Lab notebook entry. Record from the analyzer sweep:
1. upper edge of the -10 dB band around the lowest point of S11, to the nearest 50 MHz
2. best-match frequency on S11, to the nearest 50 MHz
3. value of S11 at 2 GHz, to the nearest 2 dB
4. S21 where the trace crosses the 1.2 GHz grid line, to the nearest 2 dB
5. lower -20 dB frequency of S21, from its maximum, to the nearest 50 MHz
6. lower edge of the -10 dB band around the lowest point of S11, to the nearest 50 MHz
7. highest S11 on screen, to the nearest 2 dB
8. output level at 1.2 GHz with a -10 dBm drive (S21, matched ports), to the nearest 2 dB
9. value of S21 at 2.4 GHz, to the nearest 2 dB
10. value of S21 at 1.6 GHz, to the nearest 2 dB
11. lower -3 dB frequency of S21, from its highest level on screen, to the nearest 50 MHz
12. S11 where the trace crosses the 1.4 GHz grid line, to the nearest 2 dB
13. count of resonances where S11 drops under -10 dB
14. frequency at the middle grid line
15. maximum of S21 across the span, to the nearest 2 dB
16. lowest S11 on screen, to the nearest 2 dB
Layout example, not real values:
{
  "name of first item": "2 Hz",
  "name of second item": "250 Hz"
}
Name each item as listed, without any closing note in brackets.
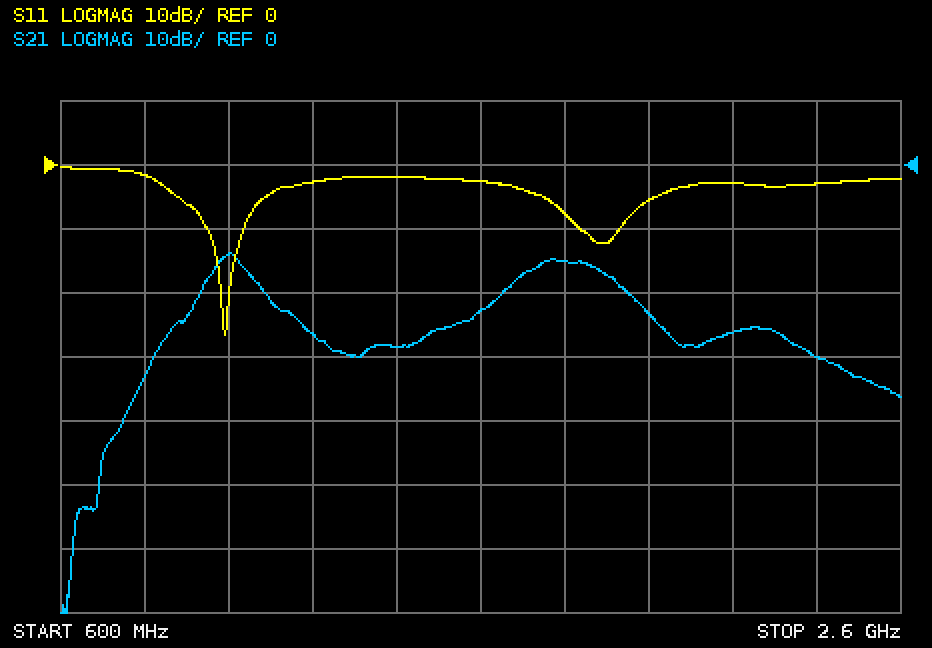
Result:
{
  "upper edge of the -10 dB band around the lowest point of S11, to the nearest 50 MHz": "1.05 GHz",
  "best-match frequency on S11, to the nearest 50 MHz": "1.00 GHz",
  "value of S11 at 2 GHz, to the nearest 2 dB": "-6 dB",
  "S21 where the trace crosses the 1.2 GHz grid line, to the nearest 2 dB": "-26 dB",
  "lower -20 dB frequency of S21, from its maximum, to the nearest 50 MHz": "800 MHz",
  "lower edge of the -10 dB band around the lowest point of S11, to the nearest 50 MHz": "950 MHz",
  "highest S11 on screen, to the nearest 2 dB": "0 dB",
  "output level at 1.2 GHz with a -10 dBm drive (S21, matched ports), to the nearest 2 dB": "-36 dBm",
  "value of S21 at 2.4 GHz, to the nearest 2 dB": "-30 dB",
  "value of S21 at 1.6 GHz, to the nearest 2 dB": "-22 dB",
  "lower -3 dB frequency of S21, from its highest level on screen, to the nearest 50 MHz": "950 MHz",
  "S11 where the trace crosses the 1.4 GHz grid line, to the nearest 2 dB": "-2 dB",
  "count of resonances where S11 drops under -10 dB": "2",
  "frequency at the middle grid line": "1.6 GHz",
  "maximum of S21 across the span, to the nearest 2 dB": "-14 dB",
  "lowest S11 on screen, to the nearest 2 dB": "-26 dB"
}
